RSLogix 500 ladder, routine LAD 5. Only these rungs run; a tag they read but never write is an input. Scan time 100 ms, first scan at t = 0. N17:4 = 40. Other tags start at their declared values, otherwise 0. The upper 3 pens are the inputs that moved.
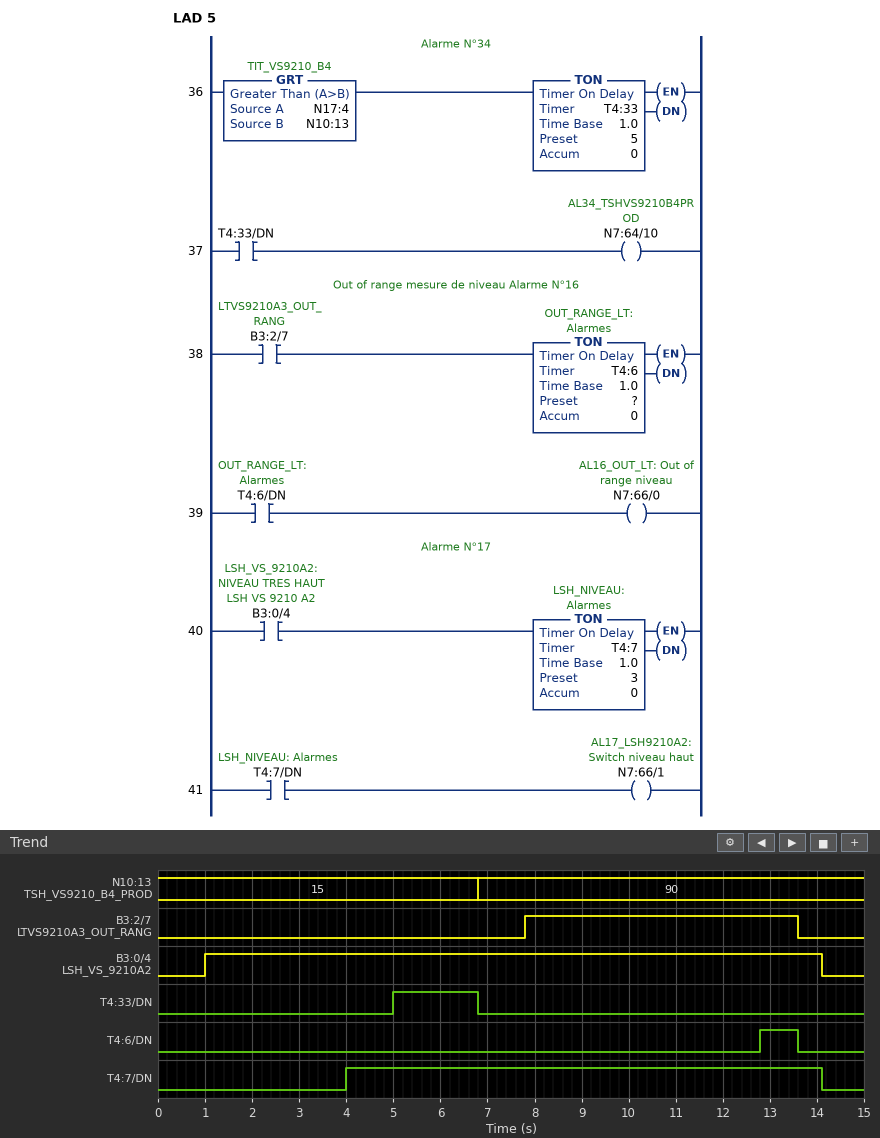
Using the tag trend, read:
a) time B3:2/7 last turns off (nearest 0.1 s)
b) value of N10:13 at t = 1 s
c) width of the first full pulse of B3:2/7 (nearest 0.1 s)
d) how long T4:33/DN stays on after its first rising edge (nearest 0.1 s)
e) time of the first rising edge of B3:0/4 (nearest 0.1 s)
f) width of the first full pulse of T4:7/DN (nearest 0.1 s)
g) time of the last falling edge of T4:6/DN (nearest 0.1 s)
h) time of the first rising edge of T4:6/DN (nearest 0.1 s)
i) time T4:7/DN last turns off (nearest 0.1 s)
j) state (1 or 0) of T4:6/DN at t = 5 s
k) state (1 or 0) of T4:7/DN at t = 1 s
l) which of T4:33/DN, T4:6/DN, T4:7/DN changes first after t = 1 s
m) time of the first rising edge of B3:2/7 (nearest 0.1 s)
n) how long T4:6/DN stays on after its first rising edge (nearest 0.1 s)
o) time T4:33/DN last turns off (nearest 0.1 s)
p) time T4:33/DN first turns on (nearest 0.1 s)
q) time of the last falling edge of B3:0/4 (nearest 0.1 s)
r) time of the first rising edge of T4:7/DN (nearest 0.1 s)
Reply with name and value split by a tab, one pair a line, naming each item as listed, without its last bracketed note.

time B3:2/7 last turns off	13.6 s
value of N10:13 at t = 1 s	15
width of the first full pulse of B3:2/7	5.8 s
how long T4:33/DN stays on after its first rising edge	1.8 s
time of the first rising edge of B3:0/4	1.0 s
width of the first full pulse of T4:7/DN	10.1 s
time of the last falling edge of T4:6/DN	13.6 s
time of the first rising edge of T4:6/DN	12.8 s
time T4:7/DN last turns off	14.1 s
state (1 or 0) of T4:6/DN at t = 5 s	0
state (1 or 0) of T4:7/DN at t = 1 s	0
which of T4:33/DN, T4:6/DN, T4:7/DN changes first after t = 1 s	T4:7/DN
time of the first rising edge of B3:2/7	7.8 s
how long T4:6/DN stays on after its first rising edge	0.8 s
time T4:33/DN last turns off	6.8 s
time T4:33/DN first turns on	5.0 s
time of the last falling edge of B3:0/4	14.1 s
time of the first rising edge of T4:7/DN	4.0 s
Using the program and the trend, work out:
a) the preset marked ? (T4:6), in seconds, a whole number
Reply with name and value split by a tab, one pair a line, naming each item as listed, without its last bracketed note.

the preset marked ? (T4:6), in seconds, a whole number	5 s
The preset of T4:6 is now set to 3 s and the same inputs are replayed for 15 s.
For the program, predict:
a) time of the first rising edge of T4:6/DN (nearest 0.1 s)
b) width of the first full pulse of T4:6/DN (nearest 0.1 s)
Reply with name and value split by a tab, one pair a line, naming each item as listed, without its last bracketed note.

time of the first rising edge of T4:6/DN	10.8 s
width of the first full pulse of T4:6/DN	2.8 s
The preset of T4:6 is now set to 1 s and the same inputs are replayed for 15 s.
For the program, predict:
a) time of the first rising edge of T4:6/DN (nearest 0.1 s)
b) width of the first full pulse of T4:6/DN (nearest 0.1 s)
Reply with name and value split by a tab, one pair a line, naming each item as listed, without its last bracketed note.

time of the first rising edge of T4:6/DN	8.8 s
width of the first full pulse of T4:6/DN	4.8 s
